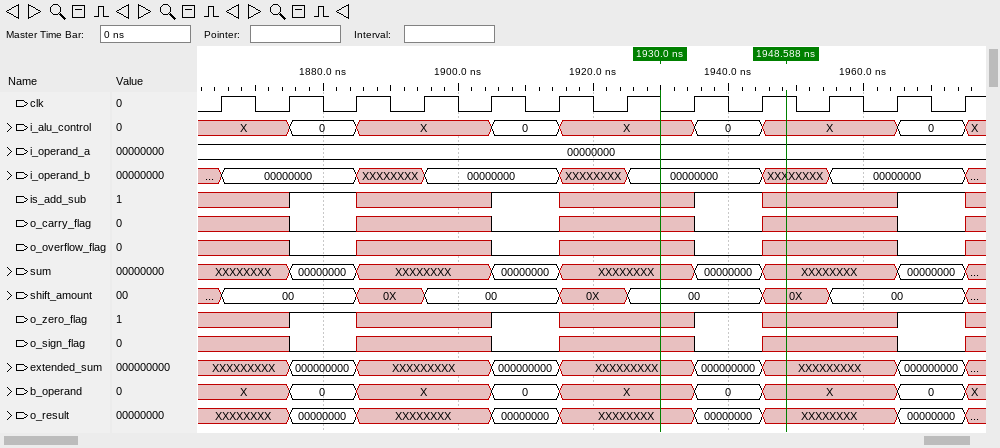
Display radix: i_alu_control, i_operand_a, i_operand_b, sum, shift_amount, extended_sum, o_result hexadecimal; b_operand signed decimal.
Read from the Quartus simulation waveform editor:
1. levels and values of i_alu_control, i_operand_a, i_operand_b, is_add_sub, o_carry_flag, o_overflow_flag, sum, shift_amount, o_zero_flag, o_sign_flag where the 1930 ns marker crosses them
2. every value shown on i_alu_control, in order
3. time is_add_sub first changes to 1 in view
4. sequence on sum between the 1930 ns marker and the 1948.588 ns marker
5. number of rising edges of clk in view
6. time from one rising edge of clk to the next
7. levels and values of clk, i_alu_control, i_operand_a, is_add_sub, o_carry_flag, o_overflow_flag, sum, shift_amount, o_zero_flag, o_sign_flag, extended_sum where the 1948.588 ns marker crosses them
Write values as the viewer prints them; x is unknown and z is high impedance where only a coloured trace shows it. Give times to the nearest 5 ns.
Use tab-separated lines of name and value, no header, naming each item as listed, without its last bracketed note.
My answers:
levels and values of i_alu_control, i_operand_a, i_operand_b, is_add_sub, o_carry_flag, o_overflow_flag, sum, shift_amount, o_zero_flag, o_sign_flag where the 1930 ns marker crosses them	i_alu_control=X, i_operand_a=00000000, i_operand_b=00000000, is_add_sub=x, o_carry_flag=x, o_overflow_flag=x, sum=XXXXXXXX, shift_amount=00, o_zero_flag=x, o_sign_flag=x
every value shown on i_alu_control, in order	X, 0, X, 0, X, 0, X, 0, X
time is_add_sub first changes to 1 in view	1875 ns
sequence on sum between the 1930 ns marker and the 1948.588 ns marker	XXXXXXXX, 00000000, XXXXXXXX
number of rising edges of clk in view	12
time from one rising edge of clk to the next	10 ns
levels and values of clk, i_alu_control, i_operand_a, is_add_sub, o_carry_flag, o_overflow_flag, sum, shift_amount, o_zero_flag, o_sign_flag, extended_sum where the 1948.588 ns marker crosses them	clk=1, i_alu_control=X, i_operand_a=00000000, is_add_sub=x, o_carry_flag=x, o_overflow_flag=x, sum=XXXXXXXX, shift_amount=0X, o_zero_flag=x, o_sign_flag=x, extended_sum=XXXXXXXXX
